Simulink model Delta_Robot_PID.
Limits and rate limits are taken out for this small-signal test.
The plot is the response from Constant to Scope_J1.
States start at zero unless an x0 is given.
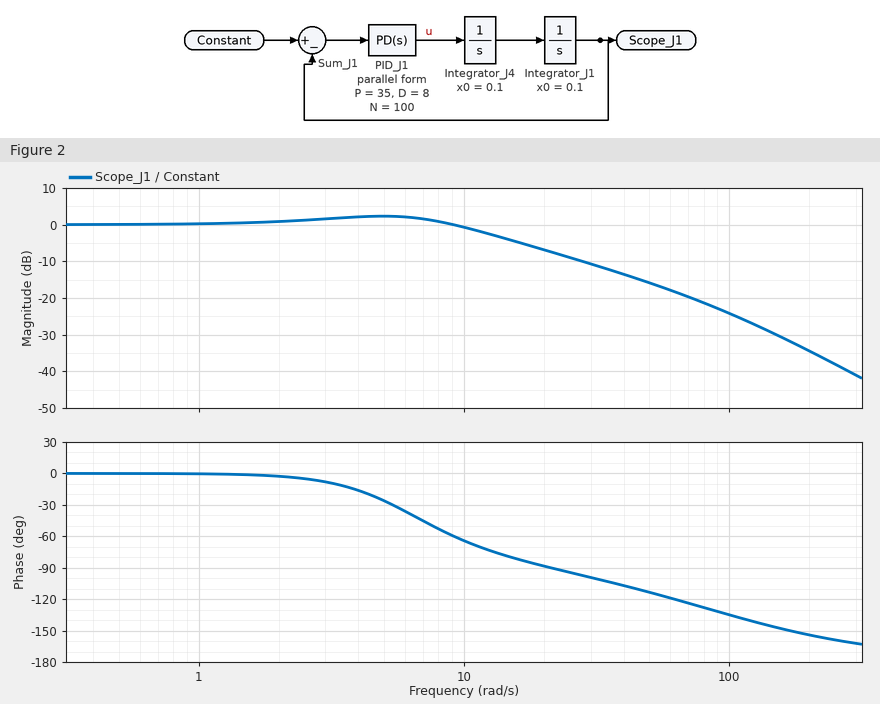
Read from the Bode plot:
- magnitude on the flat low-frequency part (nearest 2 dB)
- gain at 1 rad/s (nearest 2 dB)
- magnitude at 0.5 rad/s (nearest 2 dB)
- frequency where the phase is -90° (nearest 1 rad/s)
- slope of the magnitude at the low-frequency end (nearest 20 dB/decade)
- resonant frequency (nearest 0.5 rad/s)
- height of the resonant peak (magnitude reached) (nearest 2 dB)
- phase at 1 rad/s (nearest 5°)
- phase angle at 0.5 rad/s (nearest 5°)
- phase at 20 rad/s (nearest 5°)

0 dB
0 dB
0 dB
21 rad/s
0 dB/decade
5.0 rad/s
2 dB
0°
0°
-90°
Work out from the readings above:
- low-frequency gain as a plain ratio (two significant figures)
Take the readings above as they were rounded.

1.0
